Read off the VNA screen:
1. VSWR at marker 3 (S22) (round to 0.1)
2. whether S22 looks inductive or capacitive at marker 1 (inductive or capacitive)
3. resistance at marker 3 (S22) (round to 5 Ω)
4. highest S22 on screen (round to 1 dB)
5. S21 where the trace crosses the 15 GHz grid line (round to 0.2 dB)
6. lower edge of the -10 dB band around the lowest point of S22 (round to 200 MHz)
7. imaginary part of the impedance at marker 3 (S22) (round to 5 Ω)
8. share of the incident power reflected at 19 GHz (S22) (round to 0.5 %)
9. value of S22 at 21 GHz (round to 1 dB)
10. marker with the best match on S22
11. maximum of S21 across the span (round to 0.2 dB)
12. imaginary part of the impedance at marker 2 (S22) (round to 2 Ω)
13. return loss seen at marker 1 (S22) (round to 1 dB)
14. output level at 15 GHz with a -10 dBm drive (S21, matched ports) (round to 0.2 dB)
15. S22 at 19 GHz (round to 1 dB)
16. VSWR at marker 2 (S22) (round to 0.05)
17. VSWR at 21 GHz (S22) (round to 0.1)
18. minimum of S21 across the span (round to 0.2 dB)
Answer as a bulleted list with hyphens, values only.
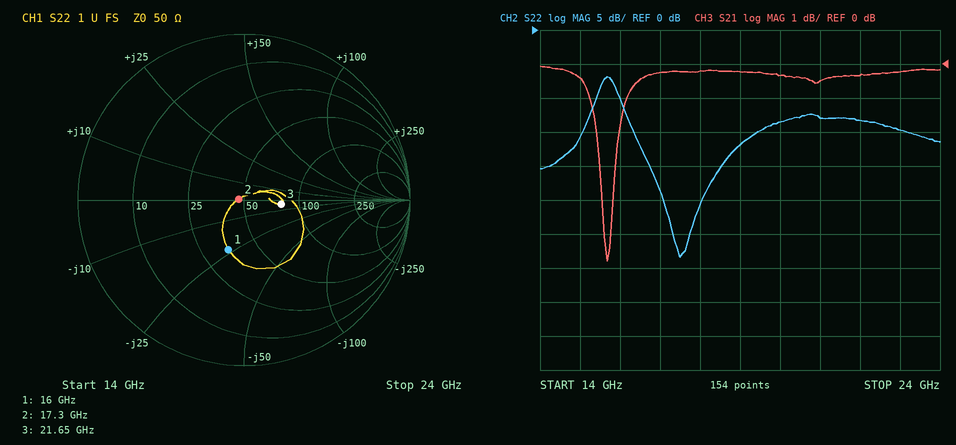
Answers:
- 1.6
- capacitive
- 80 Ω
- -7 dB
- -0.4 dB
- 16.0 GHz
- -5 Ω
- 2.0 %
- -13 dB
- marker 2
- 0.0 dB
- 0 Ω
- 10 dB
- -10.4 dBm
- -17 dB
- 1.05
- 1.6
- -5.8 dB
